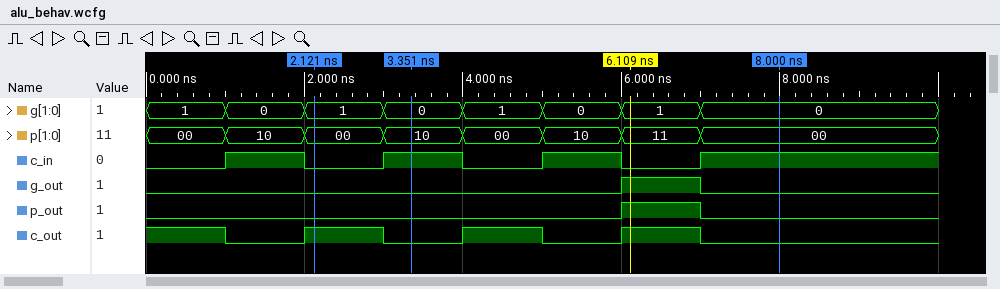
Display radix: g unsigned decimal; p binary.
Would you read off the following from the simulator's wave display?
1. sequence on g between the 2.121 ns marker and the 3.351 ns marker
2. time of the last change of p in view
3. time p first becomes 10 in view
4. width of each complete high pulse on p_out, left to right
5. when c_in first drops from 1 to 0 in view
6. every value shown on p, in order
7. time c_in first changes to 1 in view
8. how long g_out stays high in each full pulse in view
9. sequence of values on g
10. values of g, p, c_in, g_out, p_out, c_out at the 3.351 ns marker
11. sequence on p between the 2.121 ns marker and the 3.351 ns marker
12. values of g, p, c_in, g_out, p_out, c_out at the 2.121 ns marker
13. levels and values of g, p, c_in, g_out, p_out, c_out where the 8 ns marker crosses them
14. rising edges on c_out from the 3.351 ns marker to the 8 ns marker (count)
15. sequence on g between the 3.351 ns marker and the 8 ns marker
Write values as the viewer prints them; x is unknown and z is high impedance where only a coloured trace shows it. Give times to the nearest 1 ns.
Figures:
1, 0
7 ns
1 ns
1 ns
2 ns
00, 10, 00, 10, 00, 10, 11, 00
1 ns
1 ns
1, 0, 1, 0, 1, 0, 1, 0
g=0, p=10, c_in=1, g_out=0, p_out=0, c_out=0
00, 10
g=1, p=00, c_in=0, g_out=0, p_out=0, c_out=1
g=0, p=00, c_in=1, g_out=0, p_out=0, c_out=0
2
0, 1, 0, 1, 0
